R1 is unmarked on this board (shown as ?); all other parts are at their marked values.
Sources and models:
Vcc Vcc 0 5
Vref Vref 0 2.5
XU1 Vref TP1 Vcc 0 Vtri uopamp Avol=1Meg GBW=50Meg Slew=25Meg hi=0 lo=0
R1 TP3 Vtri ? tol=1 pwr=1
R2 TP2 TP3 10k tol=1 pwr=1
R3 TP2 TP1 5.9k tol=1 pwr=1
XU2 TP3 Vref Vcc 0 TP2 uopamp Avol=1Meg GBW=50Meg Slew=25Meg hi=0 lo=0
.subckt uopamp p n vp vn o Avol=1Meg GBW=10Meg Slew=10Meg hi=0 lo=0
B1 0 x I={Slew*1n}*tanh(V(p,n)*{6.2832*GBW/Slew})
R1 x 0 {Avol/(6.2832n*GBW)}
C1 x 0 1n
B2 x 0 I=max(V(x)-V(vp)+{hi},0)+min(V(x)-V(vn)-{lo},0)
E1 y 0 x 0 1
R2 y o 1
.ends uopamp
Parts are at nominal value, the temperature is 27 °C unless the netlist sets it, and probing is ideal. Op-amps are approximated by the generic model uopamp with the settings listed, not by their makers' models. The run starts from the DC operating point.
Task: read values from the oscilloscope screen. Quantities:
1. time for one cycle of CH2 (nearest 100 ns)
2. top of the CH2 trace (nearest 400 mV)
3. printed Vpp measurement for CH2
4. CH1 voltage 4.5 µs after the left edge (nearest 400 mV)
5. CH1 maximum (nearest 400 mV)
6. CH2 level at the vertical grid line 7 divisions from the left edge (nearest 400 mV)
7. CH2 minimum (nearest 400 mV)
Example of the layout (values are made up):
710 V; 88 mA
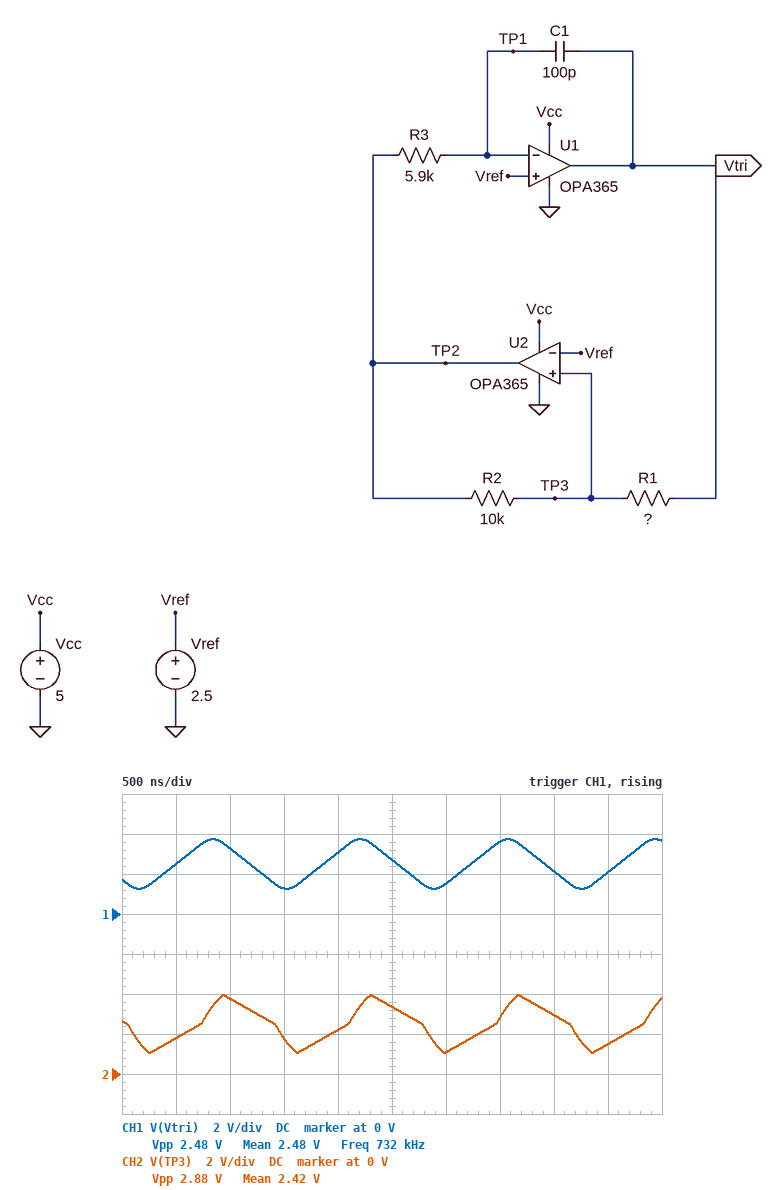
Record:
1.4 µs; 4.0 V; 2.88 V; 2.0 V; 3.6 V; 2.8 V; 1.2 V
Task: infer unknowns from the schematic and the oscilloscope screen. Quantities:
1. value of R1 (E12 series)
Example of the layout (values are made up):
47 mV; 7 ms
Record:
3.9 kΩ
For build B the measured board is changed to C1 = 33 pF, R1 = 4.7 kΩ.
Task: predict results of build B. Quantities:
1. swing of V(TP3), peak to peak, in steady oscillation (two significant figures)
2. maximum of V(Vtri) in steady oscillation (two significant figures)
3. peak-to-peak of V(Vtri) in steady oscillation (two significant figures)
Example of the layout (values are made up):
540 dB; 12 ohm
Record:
3.4 V; 4.4 V; 3.8 V
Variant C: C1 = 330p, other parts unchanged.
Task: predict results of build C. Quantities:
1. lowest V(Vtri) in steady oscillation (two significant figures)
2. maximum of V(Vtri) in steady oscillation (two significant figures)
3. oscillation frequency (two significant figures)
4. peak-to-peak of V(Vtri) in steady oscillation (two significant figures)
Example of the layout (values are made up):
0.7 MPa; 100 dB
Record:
1.4 V; 3.6 V; 290 kHz; 2.1 V
